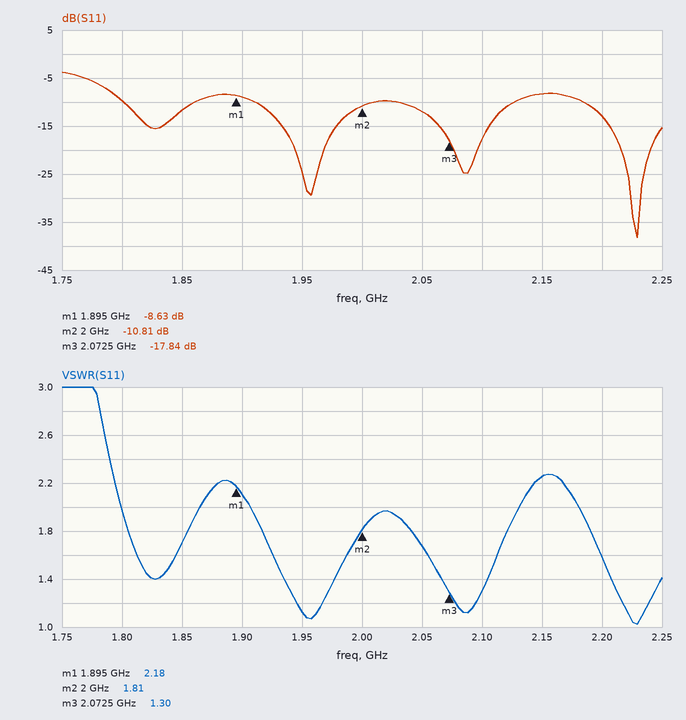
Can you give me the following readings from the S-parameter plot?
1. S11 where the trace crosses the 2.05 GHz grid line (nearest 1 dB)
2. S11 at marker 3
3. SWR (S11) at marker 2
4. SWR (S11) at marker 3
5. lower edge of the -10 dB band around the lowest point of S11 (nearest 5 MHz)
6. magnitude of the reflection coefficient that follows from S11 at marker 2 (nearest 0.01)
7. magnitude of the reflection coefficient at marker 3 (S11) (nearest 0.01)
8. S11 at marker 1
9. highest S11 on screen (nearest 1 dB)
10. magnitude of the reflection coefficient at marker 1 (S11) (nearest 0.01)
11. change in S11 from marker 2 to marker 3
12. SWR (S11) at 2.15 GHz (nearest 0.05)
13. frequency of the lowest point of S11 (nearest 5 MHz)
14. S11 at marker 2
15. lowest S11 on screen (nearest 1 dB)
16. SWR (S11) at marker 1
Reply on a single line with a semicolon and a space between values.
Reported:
-12 dB; -17.84 dB; 1.81; 1.30; 2.185 GHz; 0.29; 0.13; -8.63 dB; -4 dB; 0.37; -7.03 dB; 2.25; 2.230 GHz; -10.81 dB; -38 dB; 2.18
